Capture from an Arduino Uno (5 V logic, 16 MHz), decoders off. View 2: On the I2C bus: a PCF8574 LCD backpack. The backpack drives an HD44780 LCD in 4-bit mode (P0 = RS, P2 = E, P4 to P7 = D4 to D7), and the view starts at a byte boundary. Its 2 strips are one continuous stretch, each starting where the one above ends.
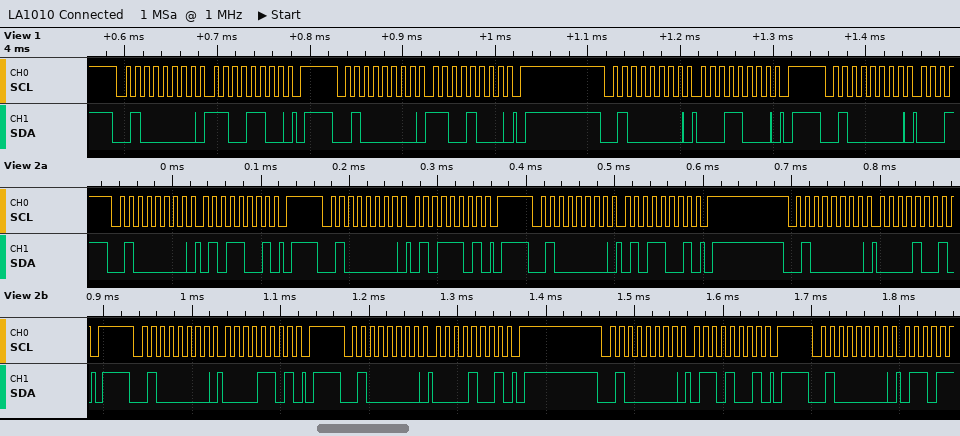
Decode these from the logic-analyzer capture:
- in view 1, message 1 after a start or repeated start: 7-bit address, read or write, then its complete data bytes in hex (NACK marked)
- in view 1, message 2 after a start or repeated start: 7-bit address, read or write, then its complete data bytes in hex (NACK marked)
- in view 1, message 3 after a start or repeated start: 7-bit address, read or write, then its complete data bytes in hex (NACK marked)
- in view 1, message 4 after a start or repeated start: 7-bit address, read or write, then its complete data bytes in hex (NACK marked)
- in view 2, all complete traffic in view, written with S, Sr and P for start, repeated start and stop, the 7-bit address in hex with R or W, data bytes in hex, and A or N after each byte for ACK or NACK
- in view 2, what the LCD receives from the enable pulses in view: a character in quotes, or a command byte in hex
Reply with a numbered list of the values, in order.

1. 0x20 write: CC
2. 0x20 write: C8
3. 0x20 write: 18
4. 0x20 write
5. S 20W A 59 A P S 20W A 5D A P S 20W A 59 A P S 20W A 09 A P S 20W A 0D A P S 20W A 09 A P S 20W A 69 A P S 20W A
6. 'P'
